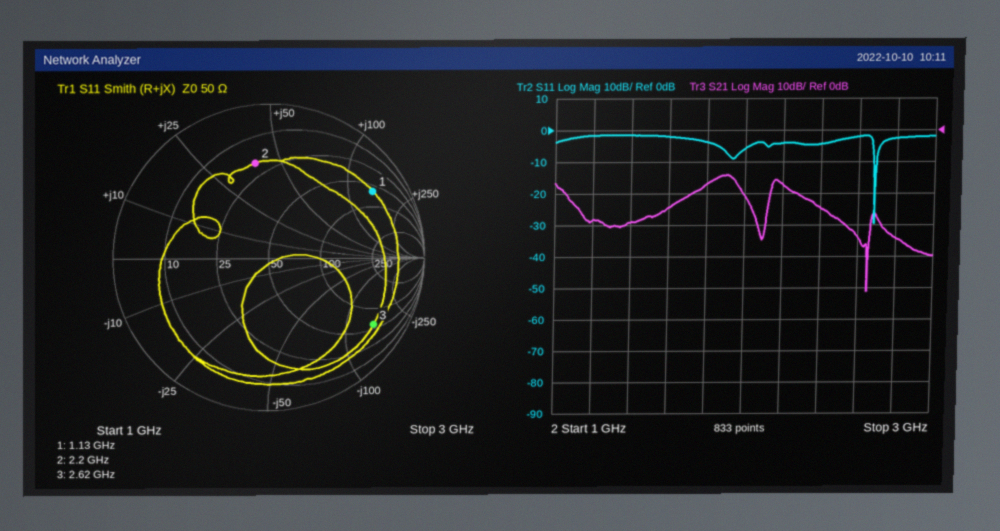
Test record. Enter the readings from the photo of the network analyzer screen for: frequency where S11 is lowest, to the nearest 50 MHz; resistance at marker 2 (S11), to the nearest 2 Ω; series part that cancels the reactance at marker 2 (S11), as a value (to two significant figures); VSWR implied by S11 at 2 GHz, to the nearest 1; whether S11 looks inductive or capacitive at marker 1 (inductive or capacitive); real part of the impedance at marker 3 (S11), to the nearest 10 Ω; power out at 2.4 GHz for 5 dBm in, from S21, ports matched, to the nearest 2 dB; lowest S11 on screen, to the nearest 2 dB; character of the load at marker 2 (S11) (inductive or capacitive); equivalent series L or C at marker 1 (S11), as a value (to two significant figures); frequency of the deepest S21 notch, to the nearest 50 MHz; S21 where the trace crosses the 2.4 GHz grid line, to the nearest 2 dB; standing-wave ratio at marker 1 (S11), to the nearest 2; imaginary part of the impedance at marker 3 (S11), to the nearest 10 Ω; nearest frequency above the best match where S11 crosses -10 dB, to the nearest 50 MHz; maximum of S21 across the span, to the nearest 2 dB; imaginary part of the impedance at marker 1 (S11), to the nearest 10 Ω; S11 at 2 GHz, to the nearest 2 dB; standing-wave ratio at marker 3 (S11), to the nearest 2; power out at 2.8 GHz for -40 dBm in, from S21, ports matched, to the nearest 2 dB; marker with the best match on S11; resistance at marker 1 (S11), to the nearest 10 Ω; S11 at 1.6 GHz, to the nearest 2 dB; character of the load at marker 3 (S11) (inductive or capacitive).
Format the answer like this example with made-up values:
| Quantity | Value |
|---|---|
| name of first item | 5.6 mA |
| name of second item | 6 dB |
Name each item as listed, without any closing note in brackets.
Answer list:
| Quantity | Value |
|---|---|
| frequency where S11 is lowest, to the nearest 50 MHz | 2.70 GHz |
| resistance at marker 2 (S11), to the nearest 2 Ω | 20 Ω |
| series part that cancels the reactance at marker 2 (S11), as a value | 1.8 pF |
| VSWR implied by S11 at 2 GHz, to the nearest 1 | 3 |
| whether S11 looks inductive or capacitive at marker 1 | inductive |
| real part of the impedance at marker 3 (S11), to the nearest 10 Ω | 60 Ω |
| power out at 2.4 GHz for 5 dBm in, from S21, ports matched, to the nearest 2 dB | -20 dBm |
| lowest S11 on screen, to the nearest 2 dB | -30 dB |
| character of the load at marker 2 (S11) | inductive |
| equivalent series L or C at marker 1 (S11), as a value | 20 nH |
| frequency of the deepest S21 notch, to the nearest 50 MHz | 2.65 GHz |
| S21 where the trace crosses the 2.4 GHz grid line, to the nearest 2 dB | -24 dB |
| standing-wave ratio at marker 1 (S11), to the nearest 2 | 8 |
| imaginary part of the impedance at marker 3 (S11), to the nearest 10 Ω | -150 Ω |
| nearest frequency above the best match where S11 crosses -10 dB, to the nearest 50 MHz | 2.70 GHz |
| maximum of S21 across the span, to the nearest 2 dB | -14 dB |
| imaginary part of the impedance at marker 1 (S11), to the nearest 10 Ω | +140 Ω |
| S11 at 2 GHz, to the nearest 2 dB | -6 dB |
| standing-wave ratio at marker 3 (S11), to the nearest 2 | 10 |
| power out at 2.8 GHz for -40 dBm in, from S21, ports matched, to the nearest 2 dB | -74 dBm |
| marker with the best match on S11 | marker 2 |
| resistance at marker 1 (S11), to the nearest 10 Ω | 60 Ω |
| S11 at 1.6 GHz, to the nearest 2 dB | -2 dB |
| character of the load at marker 3 (S11) | capacitive |
